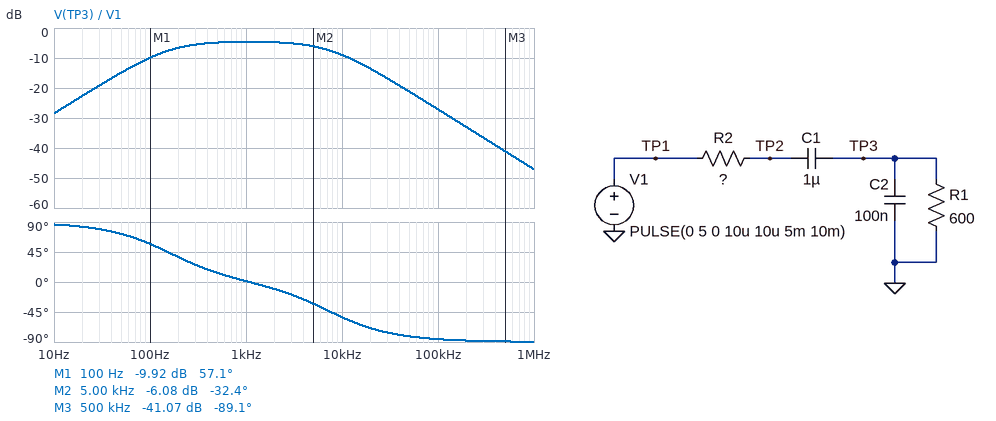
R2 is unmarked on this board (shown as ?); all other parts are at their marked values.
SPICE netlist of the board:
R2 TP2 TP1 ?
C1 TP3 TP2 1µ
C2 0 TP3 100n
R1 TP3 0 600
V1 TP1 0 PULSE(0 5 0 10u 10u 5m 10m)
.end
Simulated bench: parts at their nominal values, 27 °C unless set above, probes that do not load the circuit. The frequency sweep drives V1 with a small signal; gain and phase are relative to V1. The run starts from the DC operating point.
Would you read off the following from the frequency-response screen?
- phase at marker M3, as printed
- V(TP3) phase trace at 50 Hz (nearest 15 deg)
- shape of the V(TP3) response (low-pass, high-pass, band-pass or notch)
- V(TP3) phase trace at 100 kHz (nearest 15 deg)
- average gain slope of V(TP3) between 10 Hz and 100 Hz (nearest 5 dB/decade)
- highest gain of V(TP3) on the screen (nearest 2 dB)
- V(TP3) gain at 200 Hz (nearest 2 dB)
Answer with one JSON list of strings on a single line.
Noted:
["-89.1 deg", "75 deg", "band-pass", "-90 deg", "20 dB/decade", "-4 dB", "-6 dB"]
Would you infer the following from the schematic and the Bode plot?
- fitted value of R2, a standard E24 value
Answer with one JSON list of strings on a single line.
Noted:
["360 Ω"]
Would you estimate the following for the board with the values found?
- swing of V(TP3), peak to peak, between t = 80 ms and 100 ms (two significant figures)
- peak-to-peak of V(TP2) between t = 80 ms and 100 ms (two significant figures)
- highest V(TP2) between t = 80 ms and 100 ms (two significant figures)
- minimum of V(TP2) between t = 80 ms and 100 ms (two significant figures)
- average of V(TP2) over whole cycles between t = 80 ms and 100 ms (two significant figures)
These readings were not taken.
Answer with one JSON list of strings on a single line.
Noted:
["5.5 V", "5.0 V", "5.0 V", "12 mV", "2.5 V"]
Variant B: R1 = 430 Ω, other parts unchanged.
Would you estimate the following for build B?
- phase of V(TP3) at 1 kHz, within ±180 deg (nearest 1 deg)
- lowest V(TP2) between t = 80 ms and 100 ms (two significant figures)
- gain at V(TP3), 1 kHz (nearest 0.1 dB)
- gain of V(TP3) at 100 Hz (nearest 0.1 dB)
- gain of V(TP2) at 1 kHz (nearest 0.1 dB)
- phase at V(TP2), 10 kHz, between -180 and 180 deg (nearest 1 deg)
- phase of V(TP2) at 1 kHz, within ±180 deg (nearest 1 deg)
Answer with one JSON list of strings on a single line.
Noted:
["4 deg", "4.7 mV", "-5.8 dB", "-12.4 dB", "-4.5 dB", "-51 deg", "-14 deg"]
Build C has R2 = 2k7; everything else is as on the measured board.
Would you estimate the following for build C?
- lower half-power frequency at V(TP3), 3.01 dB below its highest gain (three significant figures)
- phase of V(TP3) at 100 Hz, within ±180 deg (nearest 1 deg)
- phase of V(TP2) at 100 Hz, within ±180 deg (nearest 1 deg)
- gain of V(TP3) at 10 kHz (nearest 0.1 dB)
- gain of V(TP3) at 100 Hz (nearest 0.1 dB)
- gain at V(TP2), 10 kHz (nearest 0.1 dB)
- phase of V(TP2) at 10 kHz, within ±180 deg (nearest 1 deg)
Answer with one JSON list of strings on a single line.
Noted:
["46.7 Hz", "24 deg", "-44 deg", "-25.0 dB", "-15.7 dB", "-24.2 dB", "-73 deg"]
